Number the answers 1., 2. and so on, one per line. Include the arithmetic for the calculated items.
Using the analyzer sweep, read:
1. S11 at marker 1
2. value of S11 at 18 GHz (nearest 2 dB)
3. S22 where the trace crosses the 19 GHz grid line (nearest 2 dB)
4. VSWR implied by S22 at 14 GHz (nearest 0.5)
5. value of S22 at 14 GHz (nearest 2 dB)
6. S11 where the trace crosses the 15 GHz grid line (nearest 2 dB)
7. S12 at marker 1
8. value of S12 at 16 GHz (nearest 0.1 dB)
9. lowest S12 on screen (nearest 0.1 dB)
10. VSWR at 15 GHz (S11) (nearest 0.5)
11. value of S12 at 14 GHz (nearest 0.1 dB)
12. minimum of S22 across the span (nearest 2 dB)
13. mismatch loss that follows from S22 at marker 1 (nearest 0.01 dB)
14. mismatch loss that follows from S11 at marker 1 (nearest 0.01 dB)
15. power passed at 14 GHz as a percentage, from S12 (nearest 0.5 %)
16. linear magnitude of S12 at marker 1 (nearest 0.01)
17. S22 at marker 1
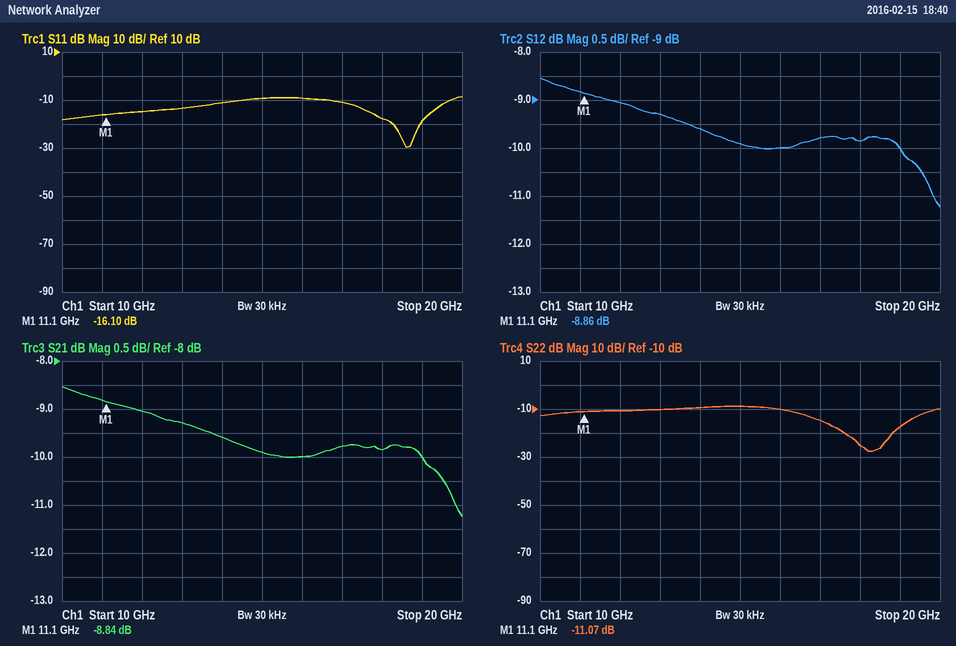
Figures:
1. -16.10 dB
2. -18 dB
3. -18 dB
4. |Γ| = 10^(-10/20) = 0.3162; VSWR = (1 + 0.3162)/(1 − 0.3162) ≈ 1.92, so 2.0 to the nearest 0.5
5. -10 dB
6. -10 dB
7. -8.86 dB
8. -10.0 dB
9. -11.2 dB
10. |Γ| = 10^(-10/20) = 0.3162; VSWR = (1 + 0.3162)/(1 − 0.3162) ≈ 1.92, so 2.0 to the nearest 0.5
11. -9.6 dB
12. -28 dB
13. −10 log10(1 − 10^(-11.07/10)) ≈ 0.35 dB
14. −10 log10(1 − 10^(-16.1/10)) ≈ 0.11 dB
15. 10^(-9.6/10) ≈ 11.0 %
16. 10^(-8.86/20) ≈ 0.36
17. -11.07 dB
